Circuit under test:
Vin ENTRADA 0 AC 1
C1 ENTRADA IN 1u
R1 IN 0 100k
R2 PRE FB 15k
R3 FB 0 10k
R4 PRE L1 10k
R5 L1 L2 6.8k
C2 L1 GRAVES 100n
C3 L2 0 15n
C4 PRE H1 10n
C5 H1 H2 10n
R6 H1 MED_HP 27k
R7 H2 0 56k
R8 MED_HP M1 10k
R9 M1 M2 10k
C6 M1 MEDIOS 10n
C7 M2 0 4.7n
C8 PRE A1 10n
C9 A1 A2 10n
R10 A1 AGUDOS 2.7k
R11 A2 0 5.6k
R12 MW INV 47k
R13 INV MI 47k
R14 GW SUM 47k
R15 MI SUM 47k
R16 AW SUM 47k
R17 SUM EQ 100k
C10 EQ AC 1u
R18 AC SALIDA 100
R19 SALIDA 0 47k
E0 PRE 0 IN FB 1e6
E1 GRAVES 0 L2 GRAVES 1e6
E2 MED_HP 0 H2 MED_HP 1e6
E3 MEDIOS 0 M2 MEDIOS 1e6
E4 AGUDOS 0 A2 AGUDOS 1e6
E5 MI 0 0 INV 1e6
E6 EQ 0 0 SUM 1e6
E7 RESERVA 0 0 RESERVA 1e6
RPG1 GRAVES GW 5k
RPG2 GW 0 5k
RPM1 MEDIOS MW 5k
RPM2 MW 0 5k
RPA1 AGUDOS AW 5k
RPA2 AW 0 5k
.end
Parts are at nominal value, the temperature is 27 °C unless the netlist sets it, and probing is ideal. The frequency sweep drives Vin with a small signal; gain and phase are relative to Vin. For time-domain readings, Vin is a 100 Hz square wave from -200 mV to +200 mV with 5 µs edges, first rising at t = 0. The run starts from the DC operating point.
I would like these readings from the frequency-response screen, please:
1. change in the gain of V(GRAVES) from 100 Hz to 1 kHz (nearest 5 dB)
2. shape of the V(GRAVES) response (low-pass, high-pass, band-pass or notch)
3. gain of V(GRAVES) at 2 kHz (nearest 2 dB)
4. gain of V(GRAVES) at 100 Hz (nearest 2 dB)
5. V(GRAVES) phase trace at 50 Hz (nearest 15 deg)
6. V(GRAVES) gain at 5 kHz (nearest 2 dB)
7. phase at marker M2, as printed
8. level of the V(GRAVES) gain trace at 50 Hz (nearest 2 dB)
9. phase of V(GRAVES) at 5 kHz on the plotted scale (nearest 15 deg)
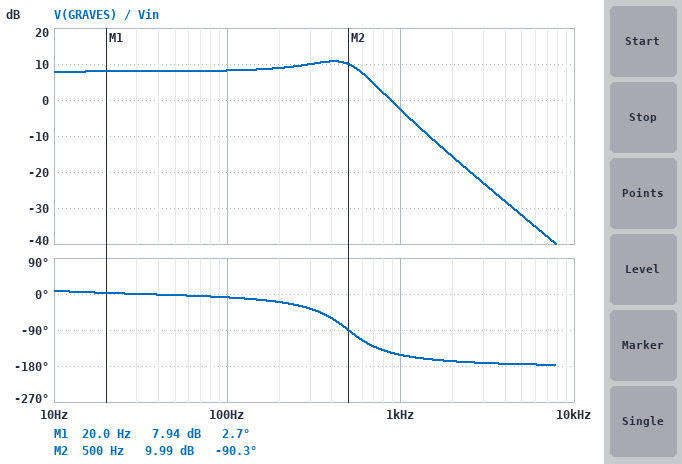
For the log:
-10 dB
low-pass
-16 dB
8 dB
0 deg
-32 dB
-90.3 deg
8 dB
-180 deg
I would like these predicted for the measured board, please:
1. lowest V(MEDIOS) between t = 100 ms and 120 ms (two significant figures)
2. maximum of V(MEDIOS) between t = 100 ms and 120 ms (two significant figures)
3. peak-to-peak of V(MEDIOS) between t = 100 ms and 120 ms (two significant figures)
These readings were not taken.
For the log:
-650 mV
650 mV
1.3 V
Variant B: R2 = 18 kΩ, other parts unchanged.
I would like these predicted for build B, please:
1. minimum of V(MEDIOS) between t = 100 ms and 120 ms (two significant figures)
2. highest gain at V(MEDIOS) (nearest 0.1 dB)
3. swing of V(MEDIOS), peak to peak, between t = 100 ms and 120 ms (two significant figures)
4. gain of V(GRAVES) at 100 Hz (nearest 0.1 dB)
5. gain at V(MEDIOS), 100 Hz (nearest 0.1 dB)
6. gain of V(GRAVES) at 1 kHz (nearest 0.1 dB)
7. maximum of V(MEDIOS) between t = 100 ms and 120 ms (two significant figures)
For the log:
-730 mV
8.8 dB
1.5 V
9.2 dB
-15.5 dB
-1.7 dB
730 mV
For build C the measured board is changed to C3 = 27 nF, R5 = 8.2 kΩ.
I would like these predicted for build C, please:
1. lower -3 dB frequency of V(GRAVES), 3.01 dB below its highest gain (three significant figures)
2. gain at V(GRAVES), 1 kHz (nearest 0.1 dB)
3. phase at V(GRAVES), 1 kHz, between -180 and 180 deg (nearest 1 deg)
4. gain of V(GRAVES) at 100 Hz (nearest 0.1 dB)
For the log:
2.08 Hz
-10.5 dB
-158 deg
8.3 dB
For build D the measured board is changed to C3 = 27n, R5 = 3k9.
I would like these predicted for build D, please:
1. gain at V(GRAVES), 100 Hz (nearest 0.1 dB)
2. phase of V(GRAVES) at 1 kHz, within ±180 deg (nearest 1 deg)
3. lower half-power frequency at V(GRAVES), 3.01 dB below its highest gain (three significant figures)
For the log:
8.1 dB
-143 deg
1.80 Hz
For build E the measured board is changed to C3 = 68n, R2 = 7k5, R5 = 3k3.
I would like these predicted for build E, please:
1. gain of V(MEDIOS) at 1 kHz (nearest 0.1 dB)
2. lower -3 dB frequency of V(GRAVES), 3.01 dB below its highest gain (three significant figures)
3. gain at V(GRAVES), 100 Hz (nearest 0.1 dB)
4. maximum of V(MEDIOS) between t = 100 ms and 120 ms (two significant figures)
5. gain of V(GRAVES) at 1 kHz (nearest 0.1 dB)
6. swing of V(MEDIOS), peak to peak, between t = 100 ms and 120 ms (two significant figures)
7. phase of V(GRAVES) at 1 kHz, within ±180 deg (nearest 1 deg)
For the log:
4.7 dB
1.57 Hz
4.2 dB
460 mV
-14.9 dB
910 mV
-144 deg
